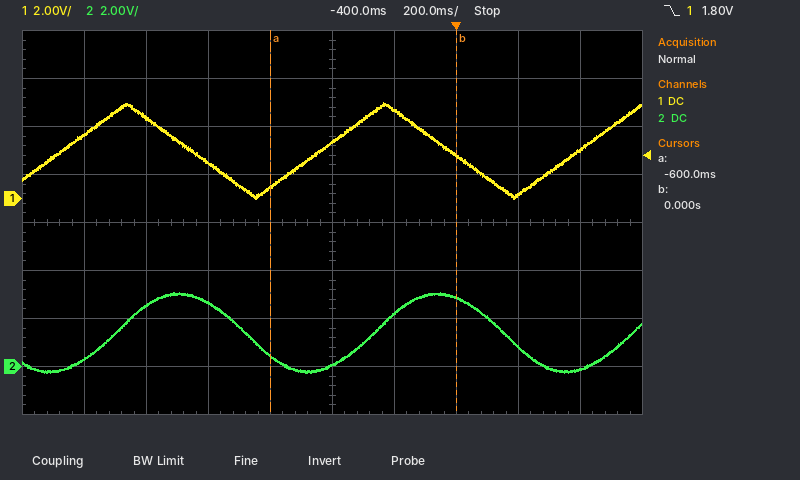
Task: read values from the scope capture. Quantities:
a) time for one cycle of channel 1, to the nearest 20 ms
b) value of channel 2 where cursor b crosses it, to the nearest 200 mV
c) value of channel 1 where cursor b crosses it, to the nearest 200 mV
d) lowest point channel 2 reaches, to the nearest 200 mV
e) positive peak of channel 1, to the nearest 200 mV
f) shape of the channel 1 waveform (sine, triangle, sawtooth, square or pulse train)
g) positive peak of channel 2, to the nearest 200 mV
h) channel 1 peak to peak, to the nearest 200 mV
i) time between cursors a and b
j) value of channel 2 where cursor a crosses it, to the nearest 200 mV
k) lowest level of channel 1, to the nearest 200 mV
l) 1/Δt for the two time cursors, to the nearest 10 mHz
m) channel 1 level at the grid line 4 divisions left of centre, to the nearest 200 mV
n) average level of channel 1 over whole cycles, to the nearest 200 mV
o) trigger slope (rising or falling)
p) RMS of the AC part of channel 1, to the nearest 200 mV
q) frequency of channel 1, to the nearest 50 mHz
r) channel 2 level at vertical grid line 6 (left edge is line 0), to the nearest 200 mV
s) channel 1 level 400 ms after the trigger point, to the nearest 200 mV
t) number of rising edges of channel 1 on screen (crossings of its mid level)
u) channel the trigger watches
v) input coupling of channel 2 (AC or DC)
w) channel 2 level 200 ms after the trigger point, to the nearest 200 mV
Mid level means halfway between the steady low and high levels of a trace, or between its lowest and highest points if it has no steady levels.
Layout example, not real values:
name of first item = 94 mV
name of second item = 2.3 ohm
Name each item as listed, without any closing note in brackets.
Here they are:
time for one cycle of channel 1, to the nearest 20 ms = 840 ms
value of channel 2 where cursor b crosses it, to the nearest 200 mV = 2.8 V
value of channel 1 where cursor b crosses it, to the nearest 200 mV = 1.8 V
lowest point channel 2 reaches, to the nearest 200 mV = -200 mV
positive peak of channel 1, to the nearest 200 mV = 4.0 V
shape of the channel 1 waveform = triangle
positive peak of channel 2, to the nearest 200 mV = 3.0 V
channel 1 peak to peak, to the nearest 200 mV = 4.0 V
time between cursors a and b = 600 ms
value of channel 2 where cursor a crosses it, to the nearest 200 mV = 400 mV
lowest level of channel 1, to the nearest 200 mV = 0.0 V
1/Δt for the two time cursors, to the nearest 10 mHz = 1.67 Hz
channel 1 level at the grid line 4 divisions left of centre, to the nearest 200 mV = 2.6 V
average level of channel 1 over whole cycles, to the nearest 200 mV = 2.0 V
trigger slope = falling
RMS of the AC part of channel 1, to the nearest 200 mV = 1.2 V
frequency of channel 1, to the nearest 50 mHz = 1.20 Hz
channel 2 level at vertical grid line 6 (left edge is line 0), to the nearest 200 mV = 2.2 V
channel 1 level 400 ms after the trigger point, to the nearest 200 mV = 2.0 V
number of rising edges of channel 1 on screen = 3
channel the trigger watches = channel 1
input coupling of channel 2 = DC
channel 2 level 200 ms after the trigger point, to the nearest 200 mV = 800 mV
